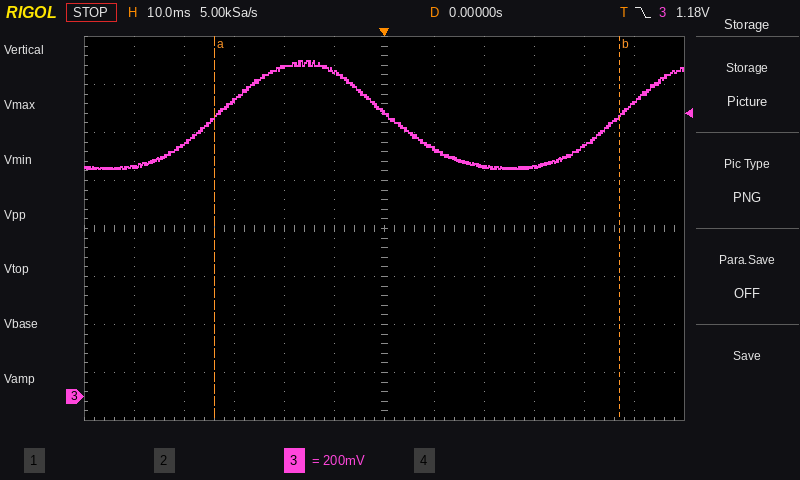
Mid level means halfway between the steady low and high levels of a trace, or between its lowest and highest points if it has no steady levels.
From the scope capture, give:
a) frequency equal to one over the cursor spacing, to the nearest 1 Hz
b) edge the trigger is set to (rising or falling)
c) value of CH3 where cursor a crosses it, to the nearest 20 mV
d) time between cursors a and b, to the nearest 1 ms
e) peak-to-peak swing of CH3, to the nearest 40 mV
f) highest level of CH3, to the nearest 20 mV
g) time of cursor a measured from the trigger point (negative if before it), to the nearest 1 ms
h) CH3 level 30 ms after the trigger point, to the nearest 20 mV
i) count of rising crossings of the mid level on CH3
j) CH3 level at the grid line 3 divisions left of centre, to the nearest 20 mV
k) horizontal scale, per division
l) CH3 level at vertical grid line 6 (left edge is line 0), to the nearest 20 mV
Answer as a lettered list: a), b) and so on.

a) 12 Hz
b) falling
c) 1.16 V
d) 81 ms
e) 440 mV
f) 1.40 V
g) -34 ms
h) 960 mV
i) 2
j) 1.24 V
k) 10 ms
l) 1.18 V
